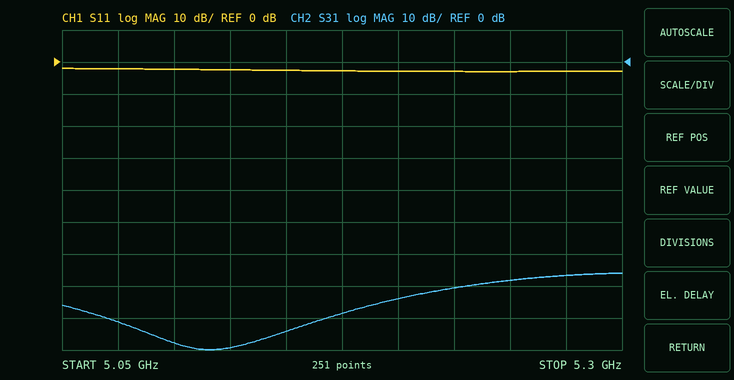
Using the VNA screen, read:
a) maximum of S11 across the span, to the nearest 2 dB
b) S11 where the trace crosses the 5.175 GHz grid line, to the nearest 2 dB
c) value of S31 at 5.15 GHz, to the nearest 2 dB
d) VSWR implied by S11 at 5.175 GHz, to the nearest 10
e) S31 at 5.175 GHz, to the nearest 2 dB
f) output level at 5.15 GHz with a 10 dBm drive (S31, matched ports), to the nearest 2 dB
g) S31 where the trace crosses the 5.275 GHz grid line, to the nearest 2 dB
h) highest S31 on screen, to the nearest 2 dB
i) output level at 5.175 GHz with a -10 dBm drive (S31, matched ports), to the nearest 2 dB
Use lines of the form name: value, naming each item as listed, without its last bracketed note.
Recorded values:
maximum of S11 across the span, to the nearest 2 dB: -2 dB
S11 where the trace crosses the 5.175 GHz grid line, to the nearest 2 dB: -2 dB
value of S31 at 5.15 GHz, to the nearest 2 dB: -84 dB
VSWR implied by S11 at 5.175 GHz, to the nearest 10: 10
S31 at 5.175 GHz, to the nearest 2 dB: -78 dB
output level at 5.15 GHz with a 10 dBm drive (S31, matched ports), to the nearest 2 dB: -74 dBm
S31 where the trace crosses the 5.275 GHz grid line, to the nearest 2 dB: -66 dB
highest S31 on screen, to the nearest 2 dB: -66 dB
output level at 5.175 GHz with a -10 dBm drive (S31, matched ports), to the nearest 2 dB: -88 dBm
